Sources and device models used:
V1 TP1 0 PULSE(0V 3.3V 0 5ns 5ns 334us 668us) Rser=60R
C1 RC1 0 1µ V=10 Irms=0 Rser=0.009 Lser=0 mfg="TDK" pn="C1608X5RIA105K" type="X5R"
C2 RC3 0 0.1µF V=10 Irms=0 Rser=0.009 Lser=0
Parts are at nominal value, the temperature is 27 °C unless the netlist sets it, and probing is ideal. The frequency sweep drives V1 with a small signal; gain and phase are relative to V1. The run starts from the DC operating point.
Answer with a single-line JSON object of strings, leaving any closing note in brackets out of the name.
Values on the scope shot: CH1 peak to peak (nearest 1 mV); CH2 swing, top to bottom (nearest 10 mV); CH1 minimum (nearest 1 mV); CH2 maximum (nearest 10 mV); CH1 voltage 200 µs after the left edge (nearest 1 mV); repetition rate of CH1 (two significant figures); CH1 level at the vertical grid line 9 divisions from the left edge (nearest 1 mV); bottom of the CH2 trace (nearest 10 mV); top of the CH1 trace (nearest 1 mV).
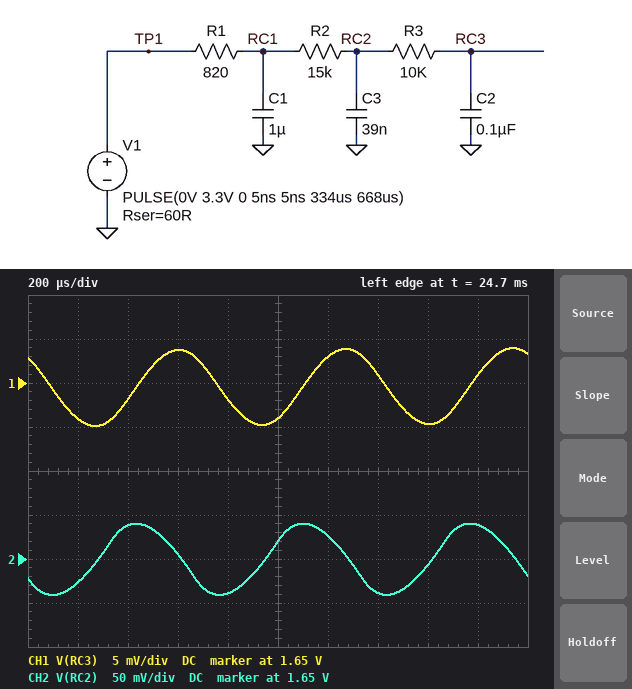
{"CH1 peak to peak": "9 mV", "CH2 swing, top to bottom": "80 mV", "CH1 minimum": "1.645 V", "CH2 maximum": "1.69 V", "CH1 voltage 200 µs after the left edge": "1.646 V", "repetition rate of CH1": "1.5 kHz", "CH1 level at the vertical grid line 9 divisions from the left edge": "1.651 V", "bottom of the CH2 trace": "1.61 V", "top of the CH1 trace": "1.654 V"}
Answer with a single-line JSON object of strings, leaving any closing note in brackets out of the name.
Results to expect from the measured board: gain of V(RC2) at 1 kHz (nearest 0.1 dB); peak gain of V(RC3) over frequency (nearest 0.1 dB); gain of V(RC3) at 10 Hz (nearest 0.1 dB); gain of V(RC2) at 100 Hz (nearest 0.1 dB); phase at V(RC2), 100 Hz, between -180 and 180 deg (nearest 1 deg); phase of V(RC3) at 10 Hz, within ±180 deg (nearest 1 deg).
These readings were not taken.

{"gain of V(RC2) at 1 kHz": "-28.3 dB", "peak gain of V(RC3) over frequency": "0 dB", "gain of V(RC3) at 10 Hz": "-0.2 dB", "gain of V(RC2) at 100 Hz": "-6.4 dB", "phase at V(RC2), 100 Hz, between -180 and 180 deg": "-65 deg", "phase of V(RC3) at 10 Hz, within ±180 deg": "-15 deg"}
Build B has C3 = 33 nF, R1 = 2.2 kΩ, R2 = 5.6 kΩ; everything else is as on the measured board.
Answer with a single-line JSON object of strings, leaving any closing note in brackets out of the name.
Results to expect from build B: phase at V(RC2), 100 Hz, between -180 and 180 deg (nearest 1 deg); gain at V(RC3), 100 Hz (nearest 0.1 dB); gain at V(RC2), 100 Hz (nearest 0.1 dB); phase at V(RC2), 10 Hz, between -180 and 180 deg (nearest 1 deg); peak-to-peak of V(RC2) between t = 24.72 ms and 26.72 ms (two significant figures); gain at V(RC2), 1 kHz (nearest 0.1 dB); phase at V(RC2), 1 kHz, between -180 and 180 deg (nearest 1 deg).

{"phase at V(RC2), 100 Hz, between -180 and 180 deg": "-72 deg", "gain at V(RC3), 100 Hz": "-8.6 dB", "gain at V(RC2), 100 Hz": "-7.1 dB", "phase at V(RC2), 10 Hz, between -180 and 180 deg": "-12 deg", "peak-to-peak of V(RC2) between t = 24.72 ms and 26.72 ms": "84 mV", "gain at V(RC2), 1 kHz": "-29.1 dB", "phase at V(RC2), 1 kHz, between -180 and 180 deg": "-124 deg"}
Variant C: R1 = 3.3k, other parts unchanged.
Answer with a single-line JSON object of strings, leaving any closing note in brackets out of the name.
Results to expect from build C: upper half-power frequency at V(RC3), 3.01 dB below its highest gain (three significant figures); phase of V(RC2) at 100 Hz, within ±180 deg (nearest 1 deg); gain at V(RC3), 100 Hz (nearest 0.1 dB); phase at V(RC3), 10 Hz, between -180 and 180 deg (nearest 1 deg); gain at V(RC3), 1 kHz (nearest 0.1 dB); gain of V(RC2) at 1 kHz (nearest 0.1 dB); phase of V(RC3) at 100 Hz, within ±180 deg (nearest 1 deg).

{"upper half-power frequency at V(RC3), 3.01 dB below its highest gain": "29.6 Hz", "phase of V(RC2) at 100 Hz, within ±180 deg": "-99 deg", "gain at V(RC3), 100 Hz": "-14.2 dB", "phase at V(RC3), 10 Hz, between -180 and 180 deg": "-24 deg", "gain at V(RC3), 1 kHz": "-55.9 dB", "gain of V(RC2) at 1 kHz": "-39.8 dB", "phase of V(RC3) at 100 Hz, within ±180 deg": "-131 deg"}
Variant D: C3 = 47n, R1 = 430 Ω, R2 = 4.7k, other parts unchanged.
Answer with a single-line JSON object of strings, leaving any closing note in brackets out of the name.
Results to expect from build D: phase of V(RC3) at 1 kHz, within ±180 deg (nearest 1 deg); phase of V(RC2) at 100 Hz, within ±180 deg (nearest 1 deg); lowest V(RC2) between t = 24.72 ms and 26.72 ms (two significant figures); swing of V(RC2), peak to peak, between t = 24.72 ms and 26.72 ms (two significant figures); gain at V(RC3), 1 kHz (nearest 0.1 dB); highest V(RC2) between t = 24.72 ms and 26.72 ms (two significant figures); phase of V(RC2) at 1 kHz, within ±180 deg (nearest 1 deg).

{"phase of V(RC3) at 1 kHz, within ±180 deg": "163 deg", "phase of V(RC2) at 100 Hz, within ±180 deg": "-35 deg", "lowest V(RC2) between t = 24.72 ms and 26.72 ms": "1.5 V", "swing of V(RC2), peak to peak, between t = 24.72 ms and 26.72 ms": "350 mV", "gain at V(RC3), 1 kHz": "-32.7 dB", "highest V(RC2) between t = 24.72 ms and 26.72 ms": "1.8 V", "phase of V(RC2) at 1 kHz, within ±180 deg": "-116 deg"}
